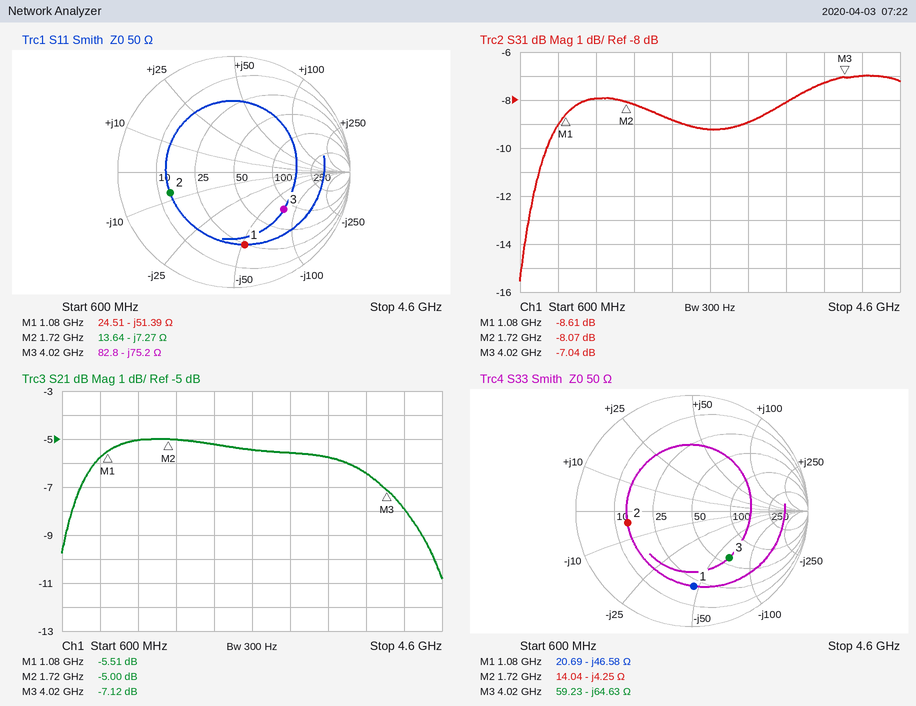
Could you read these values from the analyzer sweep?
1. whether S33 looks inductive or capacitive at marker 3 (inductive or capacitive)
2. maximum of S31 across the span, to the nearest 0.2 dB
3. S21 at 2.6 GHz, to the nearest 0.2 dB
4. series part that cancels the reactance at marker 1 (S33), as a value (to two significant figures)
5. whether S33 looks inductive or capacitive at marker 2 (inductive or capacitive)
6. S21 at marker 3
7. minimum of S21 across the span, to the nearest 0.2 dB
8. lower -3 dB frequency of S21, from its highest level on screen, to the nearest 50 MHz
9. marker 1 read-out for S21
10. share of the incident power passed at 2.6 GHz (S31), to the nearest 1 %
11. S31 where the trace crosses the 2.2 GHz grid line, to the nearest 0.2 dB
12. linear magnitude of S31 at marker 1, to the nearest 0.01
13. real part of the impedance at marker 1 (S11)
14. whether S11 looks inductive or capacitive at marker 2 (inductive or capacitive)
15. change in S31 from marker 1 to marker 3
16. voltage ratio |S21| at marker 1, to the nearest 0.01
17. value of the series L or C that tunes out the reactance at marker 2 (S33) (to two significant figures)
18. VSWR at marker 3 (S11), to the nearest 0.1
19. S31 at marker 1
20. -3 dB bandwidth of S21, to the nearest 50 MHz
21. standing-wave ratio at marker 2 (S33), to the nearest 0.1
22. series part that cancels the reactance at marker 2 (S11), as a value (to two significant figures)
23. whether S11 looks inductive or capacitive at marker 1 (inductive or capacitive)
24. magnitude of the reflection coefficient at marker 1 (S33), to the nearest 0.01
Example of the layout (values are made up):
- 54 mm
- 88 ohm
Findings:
- capacitive
- -7.0 dB
- -5.4 dB
- 6.9 nH
- capacitive
- -7.12 dB
- -10.8 dB
- 700 MHz
- -5.51 dB
- 12 %
- -8.8 dB
- 0.37
- 24.51 Ω
- capacitive
- 1.57 dB
- 0.53
- 390 pH
- 3.3
- -8.61 dB
- 3.50 GHz
- 3.6
- 670 pH
- capacitive
- 0.65
